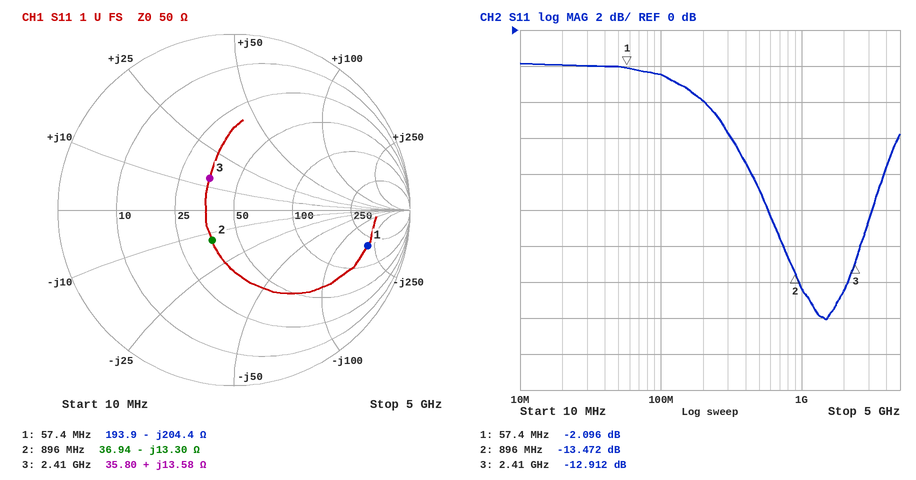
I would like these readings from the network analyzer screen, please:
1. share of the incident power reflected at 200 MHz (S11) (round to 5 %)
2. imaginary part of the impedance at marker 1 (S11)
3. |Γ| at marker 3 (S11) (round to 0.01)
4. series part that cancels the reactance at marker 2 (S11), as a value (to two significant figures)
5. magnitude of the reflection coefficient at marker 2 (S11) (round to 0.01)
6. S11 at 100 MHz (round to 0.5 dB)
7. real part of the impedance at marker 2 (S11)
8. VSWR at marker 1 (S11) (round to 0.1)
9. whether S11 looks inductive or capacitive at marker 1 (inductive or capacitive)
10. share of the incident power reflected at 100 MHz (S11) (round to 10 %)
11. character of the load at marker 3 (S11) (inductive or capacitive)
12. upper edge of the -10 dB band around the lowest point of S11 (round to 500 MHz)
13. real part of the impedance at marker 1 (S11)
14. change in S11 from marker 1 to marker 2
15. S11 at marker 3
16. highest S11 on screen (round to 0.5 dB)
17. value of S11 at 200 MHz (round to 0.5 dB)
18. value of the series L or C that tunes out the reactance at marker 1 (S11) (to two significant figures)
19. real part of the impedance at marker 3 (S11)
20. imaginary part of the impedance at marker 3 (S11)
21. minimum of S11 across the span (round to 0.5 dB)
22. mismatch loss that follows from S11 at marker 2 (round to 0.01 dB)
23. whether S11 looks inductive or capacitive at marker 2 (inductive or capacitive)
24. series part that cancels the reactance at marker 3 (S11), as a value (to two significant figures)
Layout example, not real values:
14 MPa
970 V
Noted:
40 %
-204.4 Ω
0.23
2.4 nH
0.21
-2.5 dB
36.94 Ω
8.3
capacitive
60 %
inductive
3.0 GHz
193.9 Ω
-11.376 dB
-12.912 dB
-2.0 dB
-4.0 dB
570 nH
35.80 Ω
+13.58 Ω
-16.0 dB
0.20 dB
capacitive
4.9 pF
